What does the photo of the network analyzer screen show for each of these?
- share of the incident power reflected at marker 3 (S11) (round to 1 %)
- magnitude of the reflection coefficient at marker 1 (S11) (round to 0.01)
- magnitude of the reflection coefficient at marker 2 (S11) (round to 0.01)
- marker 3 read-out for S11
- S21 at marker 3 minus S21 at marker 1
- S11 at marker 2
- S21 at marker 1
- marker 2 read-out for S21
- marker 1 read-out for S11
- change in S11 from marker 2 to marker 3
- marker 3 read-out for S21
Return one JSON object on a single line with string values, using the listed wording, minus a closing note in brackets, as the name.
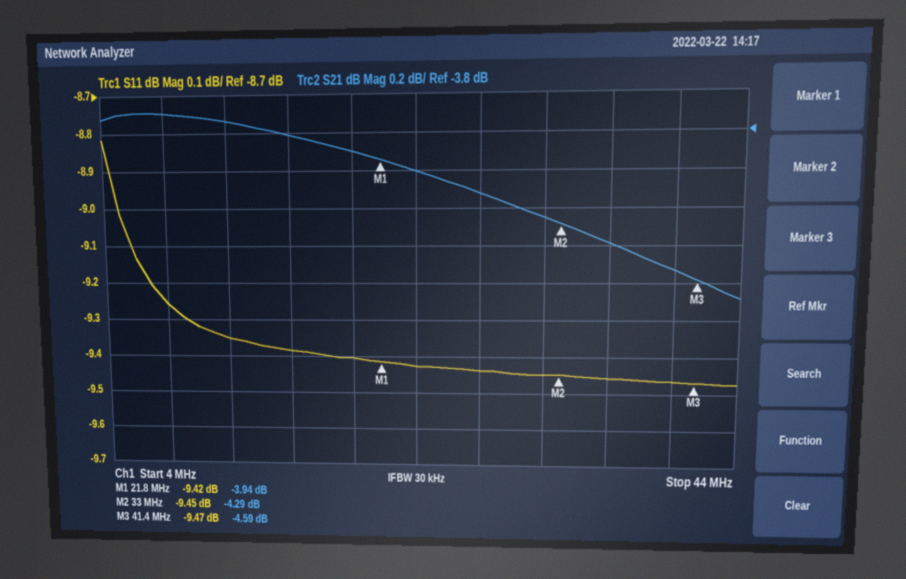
{"share of the incident power reflected at marker 3 (S11)": "11 %", "magnitude of the reflection coefficient at marker 1 (S11)": "0.34", "magnitude of the reflection coefficient at marker 2 (S11)": "0.34", "marker 3 read-out for S11": "-9.47 dB", "S21 at marker 3 minus S21 at marker 1": "-0.65 dB", "S11 at marker 2": "-9.45 dB", "S21 at marker 1": "-3.94 dB", "marker 2 read-out for S21": "-4.29 dB", "marker 1 read-out for S11": "-9.42 dB", "change in S11 from marker 2 to marker 3": "-0.02 dB", "marker 3 read-out for S21": "-4.59 dB"}
